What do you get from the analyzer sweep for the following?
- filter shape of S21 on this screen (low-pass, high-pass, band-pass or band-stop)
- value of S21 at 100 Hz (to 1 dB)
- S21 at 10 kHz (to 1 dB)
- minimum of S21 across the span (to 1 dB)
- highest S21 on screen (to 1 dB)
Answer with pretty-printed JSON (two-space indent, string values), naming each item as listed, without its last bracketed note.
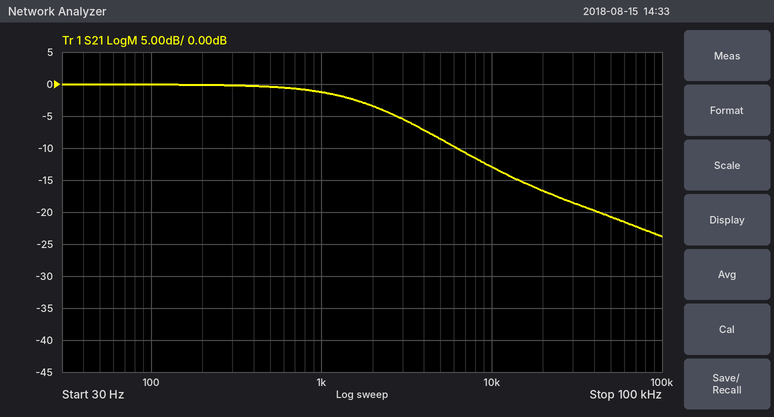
{
  "filter shape of S21 on this screen": "low-pass",
  "value of S21 at 100 Hz": "0 dB",
  "S21 at 10 kHz": "-13 dB",
  "minimum of S21 across the span": "-24 dB",
  "highest S21 on screen": "0 dB"
}
